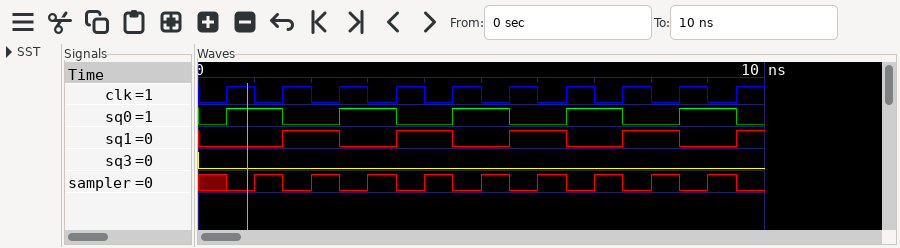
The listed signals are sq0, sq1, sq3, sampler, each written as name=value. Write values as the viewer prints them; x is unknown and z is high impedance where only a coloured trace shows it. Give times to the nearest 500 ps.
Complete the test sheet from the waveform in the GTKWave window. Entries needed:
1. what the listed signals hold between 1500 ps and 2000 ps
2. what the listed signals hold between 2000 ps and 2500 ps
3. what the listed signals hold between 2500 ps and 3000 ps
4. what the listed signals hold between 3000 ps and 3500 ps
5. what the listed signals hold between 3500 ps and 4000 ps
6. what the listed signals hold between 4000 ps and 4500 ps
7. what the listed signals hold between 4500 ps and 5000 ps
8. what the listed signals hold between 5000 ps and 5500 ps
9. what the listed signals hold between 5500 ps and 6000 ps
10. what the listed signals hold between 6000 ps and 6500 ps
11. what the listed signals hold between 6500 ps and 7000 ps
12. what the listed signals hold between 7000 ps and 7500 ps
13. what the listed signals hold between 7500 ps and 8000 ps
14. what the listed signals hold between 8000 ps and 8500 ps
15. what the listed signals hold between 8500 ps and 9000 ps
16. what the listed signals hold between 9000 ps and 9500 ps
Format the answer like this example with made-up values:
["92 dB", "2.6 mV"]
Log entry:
["sq0=0, sq1=1, sq3=0, sampler=0", "sq0=0, sq1=1, sq3=0, sampler=1", "sq0=1, sq1=0, sq3=0, sampler=0", "sq0=1, sq1=0, sq3=0, sampler=1", "sq0=0, sq1=1, sq3=0, sampler=0", "sq0=0, sq1=1, sq3=0, sampler=1", "sq0=1, sq1=0, sq3=0, sampler=0", "sq0=1, sq1=0, sq3=0, sampler=1", "sq0=0, sq1=1, sq3=0, sampler=0", "sq0=0, sq1=1, sq3=0, sampler=1", "sq0=1, sq1=0, sq3=0, sampler=0", "sq0=1, sq1=0, sq3=0, sampler=1", "sq0=0, sq1=1, sq3=0, sampler=0", "sq0=0, sq1=1, sq3=0, sampler=1", "sq0=1, sq1=0, sq3=0, sampler=0", "sq0=1, sq1=0, sq3=0, sampler=1"]
